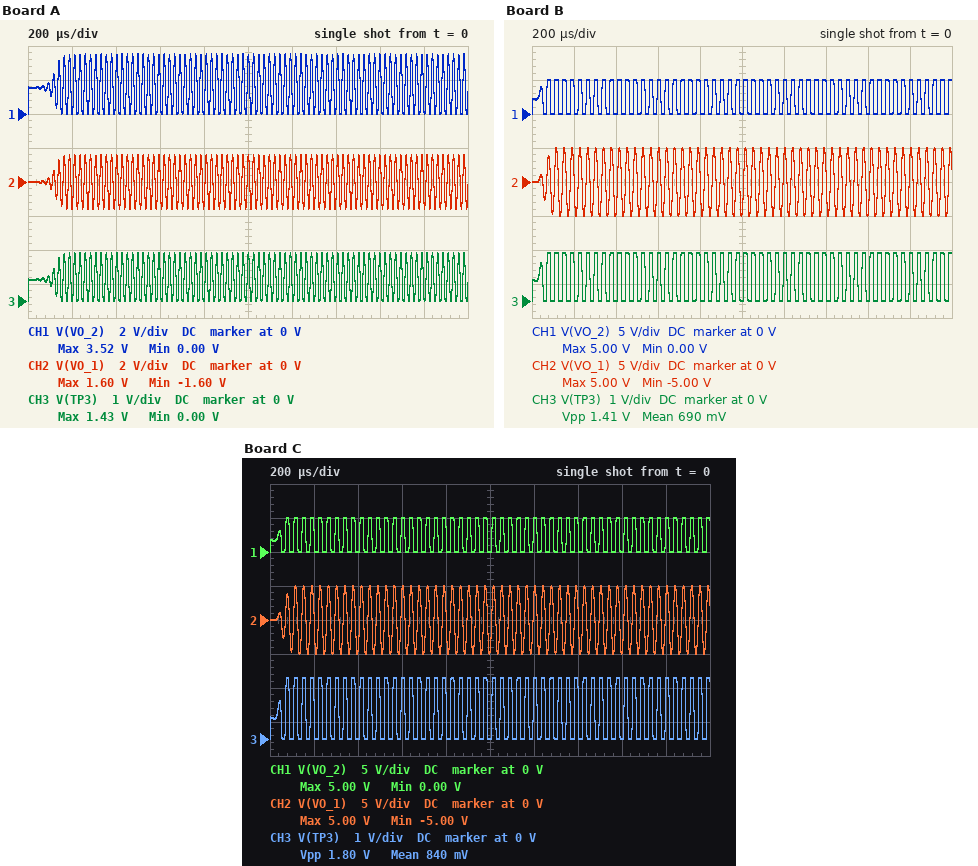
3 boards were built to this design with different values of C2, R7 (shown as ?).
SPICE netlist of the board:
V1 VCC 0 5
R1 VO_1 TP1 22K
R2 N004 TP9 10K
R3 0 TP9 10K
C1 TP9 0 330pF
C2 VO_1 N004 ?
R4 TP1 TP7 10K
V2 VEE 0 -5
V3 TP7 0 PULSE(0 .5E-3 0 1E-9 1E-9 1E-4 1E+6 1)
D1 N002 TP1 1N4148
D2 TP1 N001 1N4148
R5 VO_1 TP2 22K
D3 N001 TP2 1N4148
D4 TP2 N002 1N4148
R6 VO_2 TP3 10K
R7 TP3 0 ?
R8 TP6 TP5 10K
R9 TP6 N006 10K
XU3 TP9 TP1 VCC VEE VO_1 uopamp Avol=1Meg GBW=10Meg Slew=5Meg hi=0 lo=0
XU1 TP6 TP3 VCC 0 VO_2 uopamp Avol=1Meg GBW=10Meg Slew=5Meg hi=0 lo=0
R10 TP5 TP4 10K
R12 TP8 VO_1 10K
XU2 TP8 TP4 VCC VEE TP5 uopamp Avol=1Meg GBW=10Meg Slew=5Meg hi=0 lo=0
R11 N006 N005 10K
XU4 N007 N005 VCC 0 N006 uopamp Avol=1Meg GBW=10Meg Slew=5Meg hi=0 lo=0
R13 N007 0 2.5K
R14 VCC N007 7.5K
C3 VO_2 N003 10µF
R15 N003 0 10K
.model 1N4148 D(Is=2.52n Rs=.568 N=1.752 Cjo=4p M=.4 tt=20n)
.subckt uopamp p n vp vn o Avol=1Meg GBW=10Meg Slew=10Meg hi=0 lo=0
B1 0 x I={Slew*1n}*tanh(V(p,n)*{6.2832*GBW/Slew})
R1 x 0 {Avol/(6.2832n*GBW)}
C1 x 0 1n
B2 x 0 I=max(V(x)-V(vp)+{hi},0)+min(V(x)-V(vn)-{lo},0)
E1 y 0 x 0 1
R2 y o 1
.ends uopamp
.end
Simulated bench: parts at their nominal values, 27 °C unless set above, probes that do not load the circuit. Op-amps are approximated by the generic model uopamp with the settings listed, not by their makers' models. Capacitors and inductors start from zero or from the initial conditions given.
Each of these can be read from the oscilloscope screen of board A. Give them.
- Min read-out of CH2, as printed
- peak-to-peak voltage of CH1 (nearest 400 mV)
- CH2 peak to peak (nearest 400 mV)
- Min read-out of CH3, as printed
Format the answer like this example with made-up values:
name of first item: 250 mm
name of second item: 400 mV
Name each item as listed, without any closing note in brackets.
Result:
Min read-out of CH2, as printed: -1.60 V
peak-to-peak voltage of CH1: 3.6 V
CH2 peak to peak: 3.2 V
Min read-out of CH3, as printed: 0.00 V
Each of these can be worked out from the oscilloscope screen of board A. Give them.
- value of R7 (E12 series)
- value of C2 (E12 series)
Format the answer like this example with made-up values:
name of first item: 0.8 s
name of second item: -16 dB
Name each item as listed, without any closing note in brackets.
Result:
value of R7: 6.8 kΩ
value of C2: 390 pF
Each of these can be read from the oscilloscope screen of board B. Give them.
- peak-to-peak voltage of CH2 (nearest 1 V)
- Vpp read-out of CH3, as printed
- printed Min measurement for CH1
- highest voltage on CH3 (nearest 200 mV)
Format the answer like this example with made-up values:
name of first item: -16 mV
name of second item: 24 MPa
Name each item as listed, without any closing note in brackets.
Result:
peak-to-peak voltage of CH2: 10 V
Vpp read-out of CH3, as printed: 1.41 V
printed Min measurement for CH1: 0.00 V
highest voltage on CH3: 1.4 V
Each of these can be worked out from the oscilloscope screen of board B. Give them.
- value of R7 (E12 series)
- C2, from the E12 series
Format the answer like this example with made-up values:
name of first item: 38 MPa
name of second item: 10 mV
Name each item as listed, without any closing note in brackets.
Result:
value of R7: 3.9 kΩ
C2, from the E12 series: 1 nF
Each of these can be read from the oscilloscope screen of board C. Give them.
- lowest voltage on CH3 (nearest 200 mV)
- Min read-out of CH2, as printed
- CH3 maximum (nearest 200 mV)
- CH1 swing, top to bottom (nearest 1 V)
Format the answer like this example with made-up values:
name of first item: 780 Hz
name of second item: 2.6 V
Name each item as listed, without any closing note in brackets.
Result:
lowest voltage on CH3: 0 V
Min read-out of CH2, as printed: -5.00 V
CH3 maximum: 1.8 V
CH1 swing, top to bottom: 5 V
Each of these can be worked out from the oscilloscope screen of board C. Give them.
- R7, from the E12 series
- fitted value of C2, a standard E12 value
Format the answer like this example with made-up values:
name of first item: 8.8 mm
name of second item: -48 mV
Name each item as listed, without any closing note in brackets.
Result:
R7, from the E12 series: 5.6 kΩ
fitted value of C2, a standard E12 value: 1 nF
